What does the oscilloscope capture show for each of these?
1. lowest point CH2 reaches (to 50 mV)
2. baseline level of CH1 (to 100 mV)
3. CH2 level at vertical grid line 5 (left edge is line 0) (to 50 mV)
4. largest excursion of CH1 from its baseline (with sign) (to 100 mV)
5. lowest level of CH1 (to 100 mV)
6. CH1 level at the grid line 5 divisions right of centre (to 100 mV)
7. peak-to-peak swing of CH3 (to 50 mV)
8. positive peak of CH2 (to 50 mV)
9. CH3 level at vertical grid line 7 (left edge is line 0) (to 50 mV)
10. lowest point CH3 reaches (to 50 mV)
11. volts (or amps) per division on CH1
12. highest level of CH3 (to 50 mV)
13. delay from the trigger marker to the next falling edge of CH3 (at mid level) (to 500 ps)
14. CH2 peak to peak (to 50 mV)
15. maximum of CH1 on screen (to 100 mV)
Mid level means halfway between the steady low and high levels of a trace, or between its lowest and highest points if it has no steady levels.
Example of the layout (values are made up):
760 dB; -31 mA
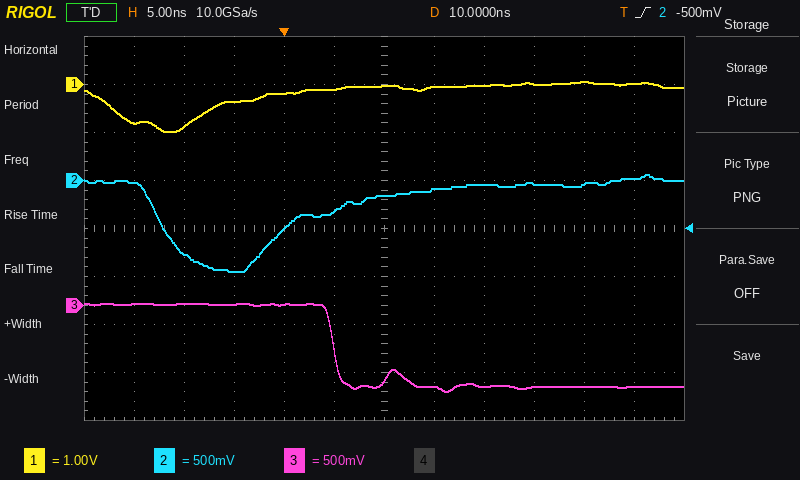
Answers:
-950 mV; 0.0 V; -300 mV; -1.0 V; -1.0 V; 0.0 V; 900 mV; 50 mV; -850 mV; -900 mV; 1 V; 0 mV; 5.0 ns; 1.00 V; 100 mV
